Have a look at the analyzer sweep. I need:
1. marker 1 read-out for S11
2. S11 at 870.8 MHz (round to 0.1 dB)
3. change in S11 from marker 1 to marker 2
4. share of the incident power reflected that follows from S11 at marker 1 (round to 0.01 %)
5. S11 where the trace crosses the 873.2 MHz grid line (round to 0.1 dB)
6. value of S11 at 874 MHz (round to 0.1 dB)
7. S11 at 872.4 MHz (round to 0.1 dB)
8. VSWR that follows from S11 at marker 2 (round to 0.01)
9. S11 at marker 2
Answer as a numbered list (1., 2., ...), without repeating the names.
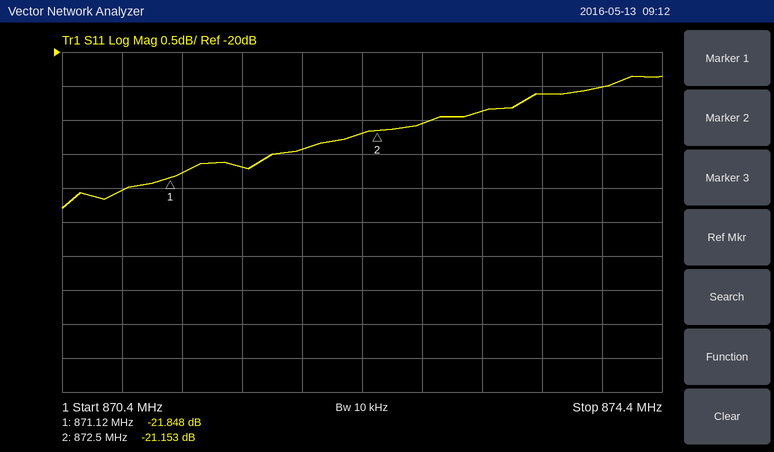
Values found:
1. -21.848 dB
2. -22.0 dB
3. 0.695 dB
4. 0.65 %
5. -20.9 dB
6. -20.5 dB
7. -21.2 dB
8. 1.19
9. -21.153 dB
